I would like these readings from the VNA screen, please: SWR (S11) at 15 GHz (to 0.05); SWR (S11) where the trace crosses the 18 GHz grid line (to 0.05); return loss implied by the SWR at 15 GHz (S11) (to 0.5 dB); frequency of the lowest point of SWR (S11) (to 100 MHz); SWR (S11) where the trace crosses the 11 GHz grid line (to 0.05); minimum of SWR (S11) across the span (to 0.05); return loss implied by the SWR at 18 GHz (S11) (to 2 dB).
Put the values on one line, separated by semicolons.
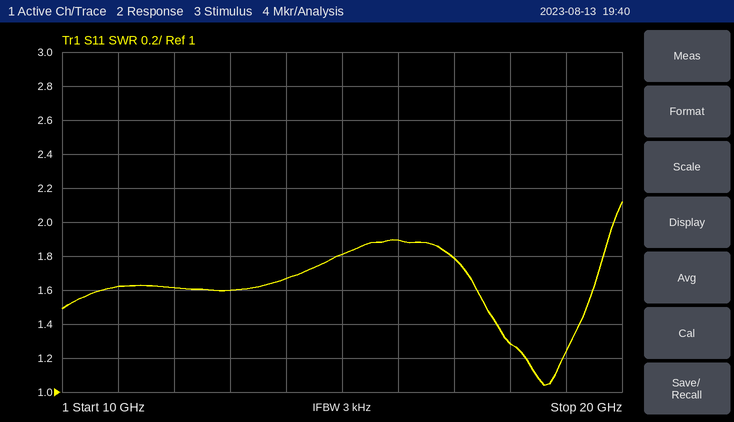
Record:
1.80; 1.30; 11.0 dB; 18.6 GHz; 1.60; 1.05; 18 dB
